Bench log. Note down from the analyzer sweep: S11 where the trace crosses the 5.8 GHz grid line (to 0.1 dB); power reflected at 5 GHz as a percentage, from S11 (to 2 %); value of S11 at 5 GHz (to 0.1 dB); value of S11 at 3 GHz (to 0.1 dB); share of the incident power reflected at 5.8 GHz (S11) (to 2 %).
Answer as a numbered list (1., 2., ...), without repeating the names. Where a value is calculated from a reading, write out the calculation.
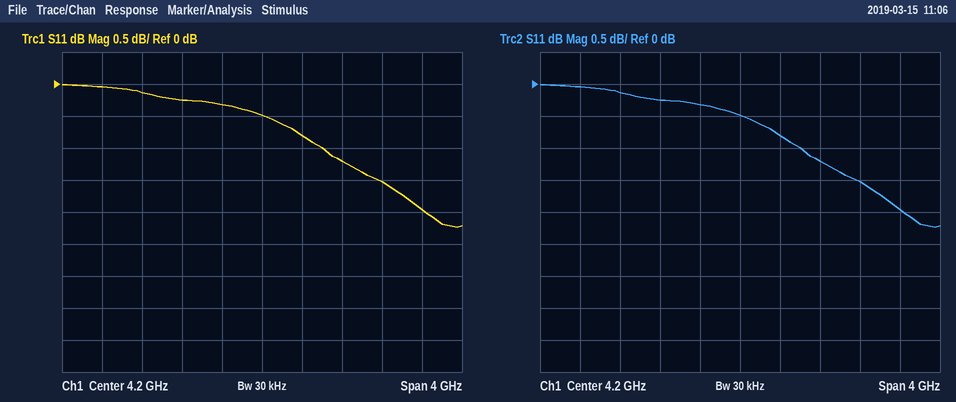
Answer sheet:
1. -2.0 dB
2. 10^(-1.2/10) ≈ 76 %
3. -1.2 dB
4. -0.1 dB
5. 10^(-2/10) ≈ 63.1 %, so 64 % to the nearest 2 %
